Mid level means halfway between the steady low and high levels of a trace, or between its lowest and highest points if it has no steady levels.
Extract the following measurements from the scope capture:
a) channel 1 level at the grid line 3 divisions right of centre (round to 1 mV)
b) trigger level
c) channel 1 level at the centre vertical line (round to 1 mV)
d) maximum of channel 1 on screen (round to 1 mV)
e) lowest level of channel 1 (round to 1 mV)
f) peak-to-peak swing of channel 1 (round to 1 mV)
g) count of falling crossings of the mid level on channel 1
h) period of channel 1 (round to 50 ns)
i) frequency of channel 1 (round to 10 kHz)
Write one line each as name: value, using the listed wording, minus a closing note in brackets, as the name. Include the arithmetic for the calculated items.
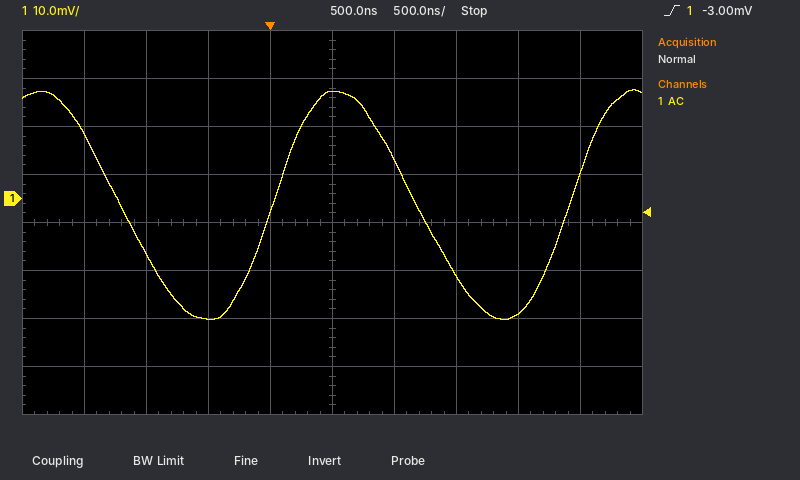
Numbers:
channel 1 level at the grid line 3 divisions right of centre: -24 mV
trigger level: -3.00 mV
channel 1 level at the centre vertical line: 22 mV
maximum of channel 1 on screen: 23 mV
lowest level of channel 1: -25 mV
peak-to-peak swing of channel 1: 23 mV − (-25 mV) = 48 mV
count of falling crossings of the mid level on channel 1: 2
period of channel 1: 2.40 µs
frequency of channel 1: 1 / 2.40 µs ≈ 417 kHz, so 420 kHz to the nearest 10 kHz
